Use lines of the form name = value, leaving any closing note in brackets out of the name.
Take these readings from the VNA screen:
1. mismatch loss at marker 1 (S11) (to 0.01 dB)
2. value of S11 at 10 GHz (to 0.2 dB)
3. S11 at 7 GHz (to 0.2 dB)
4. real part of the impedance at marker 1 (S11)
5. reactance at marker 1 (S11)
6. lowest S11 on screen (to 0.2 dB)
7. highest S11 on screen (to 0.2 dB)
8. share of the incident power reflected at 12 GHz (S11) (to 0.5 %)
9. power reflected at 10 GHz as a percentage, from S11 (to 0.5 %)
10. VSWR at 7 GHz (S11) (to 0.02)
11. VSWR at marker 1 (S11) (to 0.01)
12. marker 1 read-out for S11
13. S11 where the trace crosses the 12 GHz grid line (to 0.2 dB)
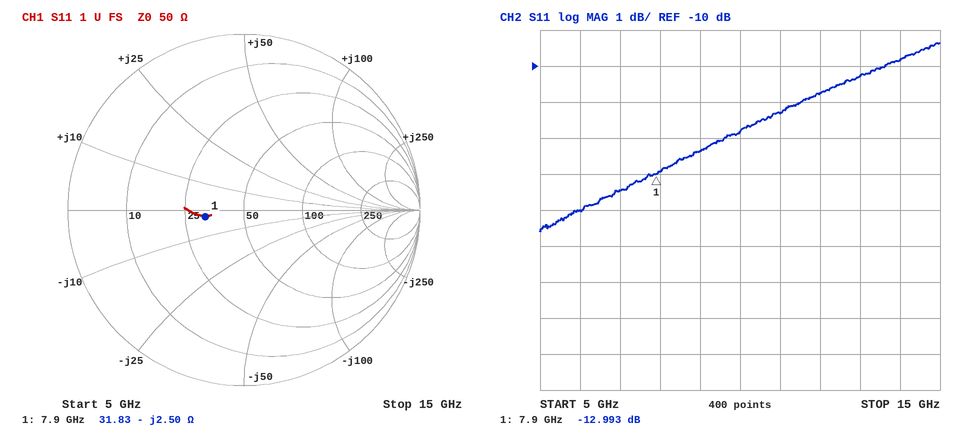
mismatch loss at marker 1 (S11) = 0.22 dB
value of S11 at 10 GHz = -11.8 dB
S11 at 7 GHz = -13.4 dB
real part of the impedance at marker 1 = 31.83 Ω
reactance at marker 1 = -2.50 Ω
lowest S11 on screen = -14.6 dB
highest S11 on screen = -9.4 dB
share of the incident power reflected at 12 GHz (S11) = 8.5 %
power reflected at 10 GHz as a percentage, from S11 = 6.5 %
VSWR at 7 GHz (S11) = 1.54
VSWR at marker 1 (S11) = 1.58
marker 1 read-out for S11 = -12.993 dB
S11 where the trace crosses the 12 GHz grid line = -10.8 dB
